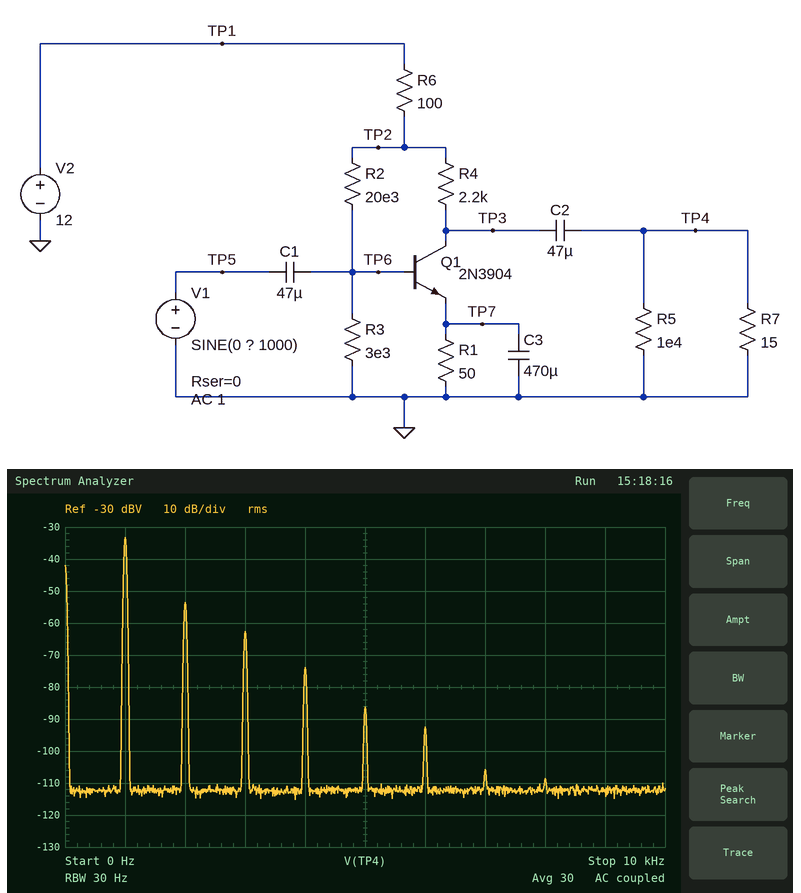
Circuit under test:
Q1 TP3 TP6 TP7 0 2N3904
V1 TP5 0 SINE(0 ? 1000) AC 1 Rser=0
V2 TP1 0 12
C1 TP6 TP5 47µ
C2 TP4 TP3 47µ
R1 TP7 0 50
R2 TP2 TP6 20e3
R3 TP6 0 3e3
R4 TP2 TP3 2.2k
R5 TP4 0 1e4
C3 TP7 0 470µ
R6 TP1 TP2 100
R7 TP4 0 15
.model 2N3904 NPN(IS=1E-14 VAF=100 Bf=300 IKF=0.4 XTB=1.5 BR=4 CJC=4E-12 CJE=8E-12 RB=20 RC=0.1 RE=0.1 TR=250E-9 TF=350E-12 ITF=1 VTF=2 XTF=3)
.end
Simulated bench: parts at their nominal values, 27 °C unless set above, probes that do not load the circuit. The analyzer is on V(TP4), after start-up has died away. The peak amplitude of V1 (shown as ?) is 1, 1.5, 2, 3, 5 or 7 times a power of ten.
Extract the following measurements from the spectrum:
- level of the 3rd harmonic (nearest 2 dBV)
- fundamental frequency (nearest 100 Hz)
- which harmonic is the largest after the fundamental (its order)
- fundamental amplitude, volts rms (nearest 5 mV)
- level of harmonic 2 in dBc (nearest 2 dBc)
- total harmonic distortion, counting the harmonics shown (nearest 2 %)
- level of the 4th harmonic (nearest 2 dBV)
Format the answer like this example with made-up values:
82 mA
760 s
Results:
-62 dBV
1.0 kHz
2
20 mV
-20 dBc
10 %
-74 dBV
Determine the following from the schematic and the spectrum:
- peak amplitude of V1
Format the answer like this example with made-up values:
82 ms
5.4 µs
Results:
20 mV
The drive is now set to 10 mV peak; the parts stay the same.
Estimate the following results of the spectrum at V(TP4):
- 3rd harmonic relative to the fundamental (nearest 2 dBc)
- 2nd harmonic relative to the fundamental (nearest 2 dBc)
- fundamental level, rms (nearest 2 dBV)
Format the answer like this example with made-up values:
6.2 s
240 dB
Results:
-44 dBc
-22 dBc
-40 dBV
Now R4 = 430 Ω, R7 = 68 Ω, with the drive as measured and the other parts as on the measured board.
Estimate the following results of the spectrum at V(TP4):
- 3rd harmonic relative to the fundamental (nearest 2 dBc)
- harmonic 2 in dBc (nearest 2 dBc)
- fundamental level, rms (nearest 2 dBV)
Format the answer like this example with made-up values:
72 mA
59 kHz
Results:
-38 dBc
-16 dBc
-10 dBV
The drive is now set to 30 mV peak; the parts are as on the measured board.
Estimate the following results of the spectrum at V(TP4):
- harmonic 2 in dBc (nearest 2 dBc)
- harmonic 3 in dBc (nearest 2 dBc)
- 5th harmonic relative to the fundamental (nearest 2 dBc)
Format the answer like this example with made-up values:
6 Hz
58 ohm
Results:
-24 dBc
-22 dBc
-38 dBc
